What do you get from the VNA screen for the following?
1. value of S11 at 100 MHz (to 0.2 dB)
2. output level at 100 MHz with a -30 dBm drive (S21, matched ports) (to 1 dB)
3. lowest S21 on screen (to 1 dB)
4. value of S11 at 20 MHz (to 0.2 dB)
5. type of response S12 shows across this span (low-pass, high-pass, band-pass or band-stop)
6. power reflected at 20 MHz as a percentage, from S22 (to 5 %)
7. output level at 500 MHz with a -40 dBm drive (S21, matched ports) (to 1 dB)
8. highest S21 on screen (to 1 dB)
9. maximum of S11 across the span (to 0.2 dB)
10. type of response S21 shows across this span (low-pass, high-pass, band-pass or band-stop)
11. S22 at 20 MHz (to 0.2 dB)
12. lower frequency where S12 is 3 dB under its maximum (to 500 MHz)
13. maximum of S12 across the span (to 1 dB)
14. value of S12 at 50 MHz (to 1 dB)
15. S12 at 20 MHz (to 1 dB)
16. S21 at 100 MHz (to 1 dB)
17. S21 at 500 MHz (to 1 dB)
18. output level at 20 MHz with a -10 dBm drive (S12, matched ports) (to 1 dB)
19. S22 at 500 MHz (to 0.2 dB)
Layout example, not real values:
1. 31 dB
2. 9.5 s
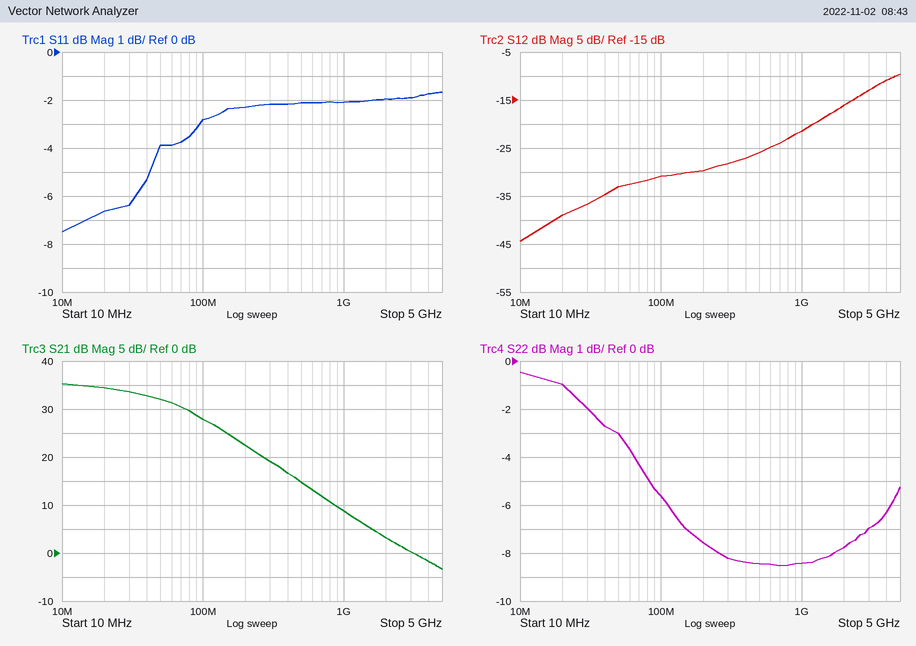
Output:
1. -2.8 dB
2. -2 dBm
3. -3 dB
4. -6.6 dB
5. high-pass
6. 80 %
7. -25 dBm
8. 35 dB
9. -1.6 dB
10. low-pass
11. -1.0 dB
12. 3.0 GHz
13. -10 dB
14. -33 dB
15. -39 dB
16. 28 dB
17. 15 dB
18. -49 dBm
19. -8.4 dB
